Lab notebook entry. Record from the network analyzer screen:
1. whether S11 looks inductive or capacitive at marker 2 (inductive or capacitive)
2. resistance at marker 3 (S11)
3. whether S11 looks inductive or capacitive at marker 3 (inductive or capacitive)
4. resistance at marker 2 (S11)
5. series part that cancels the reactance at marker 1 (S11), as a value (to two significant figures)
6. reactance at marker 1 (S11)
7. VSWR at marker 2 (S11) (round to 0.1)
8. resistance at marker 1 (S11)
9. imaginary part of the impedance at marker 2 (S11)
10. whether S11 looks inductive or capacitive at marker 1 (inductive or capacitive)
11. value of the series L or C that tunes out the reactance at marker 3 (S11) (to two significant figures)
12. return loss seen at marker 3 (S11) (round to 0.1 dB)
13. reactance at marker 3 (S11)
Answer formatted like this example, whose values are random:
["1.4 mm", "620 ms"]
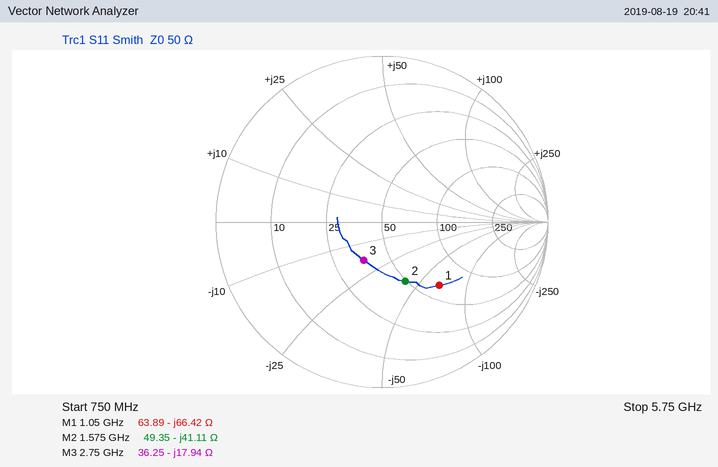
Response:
["capacitive", "36.25 Ω", "capacitive", "49.35 Ω", "10 nH", "-66.42 Ω", "2.2", "63.89 Ω", "-41.11 Ω", "capacitive", "1.0 nH", "11.8 dB", "-17.94 Ω"]
